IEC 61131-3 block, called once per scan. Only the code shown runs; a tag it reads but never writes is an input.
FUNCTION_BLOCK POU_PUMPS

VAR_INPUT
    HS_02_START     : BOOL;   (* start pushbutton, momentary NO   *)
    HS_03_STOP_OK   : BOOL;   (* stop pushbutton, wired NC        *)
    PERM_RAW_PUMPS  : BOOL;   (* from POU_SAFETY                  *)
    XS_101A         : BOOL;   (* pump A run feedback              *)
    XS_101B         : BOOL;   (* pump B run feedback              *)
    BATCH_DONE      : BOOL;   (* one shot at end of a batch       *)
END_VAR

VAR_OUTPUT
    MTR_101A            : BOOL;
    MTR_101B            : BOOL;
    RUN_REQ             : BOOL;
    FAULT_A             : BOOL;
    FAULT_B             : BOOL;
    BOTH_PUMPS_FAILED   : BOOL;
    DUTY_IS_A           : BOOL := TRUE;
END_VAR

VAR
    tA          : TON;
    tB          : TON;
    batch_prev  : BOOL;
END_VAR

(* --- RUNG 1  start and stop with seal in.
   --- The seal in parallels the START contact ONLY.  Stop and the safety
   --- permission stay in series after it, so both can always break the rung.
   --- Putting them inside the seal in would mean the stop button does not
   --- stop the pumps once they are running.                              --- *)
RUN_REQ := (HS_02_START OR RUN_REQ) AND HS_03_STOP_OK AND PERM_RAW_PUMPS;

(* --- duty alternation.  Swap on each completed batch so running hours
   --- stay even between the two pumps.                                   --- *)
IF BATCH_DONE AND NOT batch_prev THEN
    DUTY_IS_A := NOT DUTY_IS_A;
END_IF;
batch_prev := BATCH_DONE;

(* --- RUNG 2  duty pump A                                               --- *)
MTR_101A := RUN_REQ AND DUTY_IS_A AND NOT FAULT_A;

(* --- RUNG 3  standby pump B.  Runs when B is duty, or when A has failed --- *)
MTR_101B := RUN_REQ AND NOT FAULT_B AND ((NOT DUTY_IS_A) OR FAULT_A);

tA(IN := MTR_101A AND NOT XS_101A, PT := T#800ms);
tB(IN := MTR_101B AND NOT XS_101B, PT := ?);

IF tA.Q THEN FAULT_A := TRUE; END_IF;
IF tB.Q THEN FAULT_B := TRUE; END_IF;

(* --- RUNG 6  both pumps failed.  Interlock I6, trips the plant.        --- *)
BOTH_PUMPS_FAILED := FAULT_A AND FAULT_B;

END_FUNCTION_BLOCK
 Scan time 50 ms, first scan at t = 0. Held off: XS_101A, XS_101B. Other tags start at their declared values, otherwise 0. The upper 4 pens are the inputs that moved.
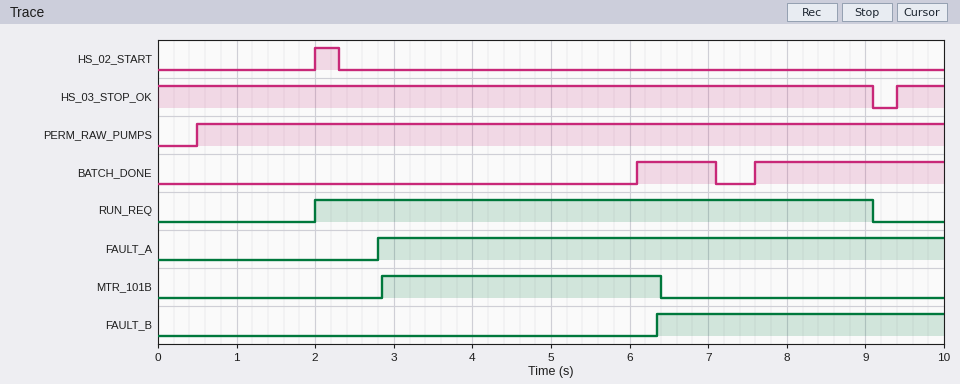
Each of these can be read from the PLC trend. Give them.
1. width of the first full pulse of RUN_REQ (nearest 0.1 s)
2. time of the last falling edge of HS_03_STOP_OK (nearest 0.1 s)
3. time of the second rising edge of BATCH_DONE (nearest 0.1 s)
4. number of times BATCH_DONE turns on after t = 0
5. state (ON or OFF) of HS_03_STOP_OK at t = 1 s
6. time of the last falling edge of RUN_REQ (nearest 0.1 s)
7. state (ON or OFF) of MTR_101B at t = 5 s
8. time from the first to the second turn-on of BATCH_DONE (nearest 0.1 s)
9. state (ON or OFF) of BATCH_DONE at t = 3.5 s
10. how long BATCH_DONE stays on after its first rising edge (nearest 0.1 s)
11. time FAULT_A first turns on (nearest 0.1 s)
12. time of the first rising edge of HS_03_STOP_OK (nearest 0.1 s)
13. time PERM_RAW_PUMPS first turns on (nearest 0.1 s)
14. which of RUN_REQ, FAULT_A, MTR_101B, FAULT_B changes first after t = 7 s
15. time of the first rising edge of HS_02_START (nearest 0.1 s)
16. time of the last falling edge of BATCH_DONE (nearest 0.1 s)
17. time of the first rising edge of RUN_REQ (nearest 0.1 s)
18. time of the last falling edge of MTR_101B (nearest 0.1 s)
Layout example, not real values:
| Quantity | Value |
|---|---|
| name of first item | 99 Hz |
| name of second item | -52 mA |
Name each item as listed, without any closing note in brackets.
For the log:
| Quantity | Value |
|---|---|
| width of the first full pulse of RUN_REQ | 7.1 s |
| time of the last falling edge of HS_03_STOP_OK | 9.1 s |
| time of the second rising edge of BATCH_DONE | 7.6 s |
| number of times BATCH_DONE turns on after t = 0 | 2 |
| state (ON or OFF) of HS_03_STOP_OK at t = 1 s | ON |
| time of the last falling edge of RUN_REQ | 9.1 s |
| state (ON or OFF) of MTR_101B at t = 5 s | ON |
| time from the first to the second turn-on of BATCH_DONE | 1.5 s |
| state (ON or OFF) of BATCH_DONE at t = 3.5 s | OFF |
| how long BATCH_DONE stays on after its first rising edge | 1.0 s |
| time FAULT_A first turns on | 2.8 s |
| time of the first rising edge of HS_03_STOP_OK | 9.4 s |
| time PERM_RAW_PUMPS first turns on | 0.5 s |
| which of RUN_REQ, FAULT_A, MTR_101B, FAULT_B changes first after t = 7 s | RUN_REQ |
| time of the first rising edge of HS_02_START | 2.0 s |
| time of the last falling edge of BATCH_DONE | 7.1 s |
| time of the first rising edge of RUN_REQ | 2.0 s |
| time of the last falling edge of MTR_101B | 6.4 s |
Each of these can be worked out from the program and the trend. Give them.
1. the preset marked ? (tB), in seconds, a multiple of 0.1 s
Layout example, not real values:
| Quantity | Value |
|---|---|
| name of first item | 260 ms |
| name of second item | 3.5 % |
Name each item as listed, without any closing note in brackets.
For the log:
| Quantity | Value |
|---|---|
| the preset marked ? (tB), in seconds, a multiple of 0.1 s | 3.5 s |
